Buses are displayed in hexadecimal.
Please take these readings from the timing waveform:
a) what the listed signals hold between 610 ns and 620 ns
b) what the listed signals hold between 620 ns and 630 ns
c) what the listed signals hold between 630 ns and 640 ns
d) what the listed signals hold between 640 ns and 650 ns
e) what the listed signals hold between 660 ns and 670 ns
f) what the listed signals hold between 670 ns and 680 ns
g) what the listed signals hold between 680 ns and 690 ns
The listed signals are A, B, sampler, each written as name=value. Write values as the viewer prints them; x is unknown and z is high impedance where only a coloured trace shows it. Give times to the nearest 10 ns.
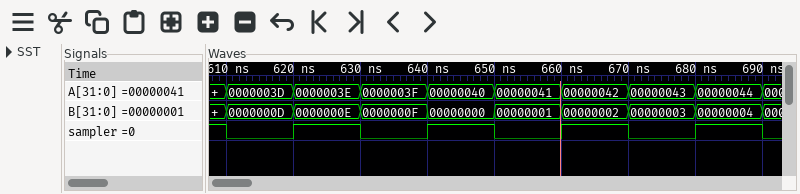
A=0000003D, B=0000000D, sampler=0
A=0000003E, B=0000000E, sampler=1
A=0000003F, B=0000000F, sampler=0
A=00000040, B=00000000, sampler=1
A=00000042, B=00000002, sampler=1
A=00000043, B=00000003, sampler=0
A=00000044, B=00000004, sampler=1
